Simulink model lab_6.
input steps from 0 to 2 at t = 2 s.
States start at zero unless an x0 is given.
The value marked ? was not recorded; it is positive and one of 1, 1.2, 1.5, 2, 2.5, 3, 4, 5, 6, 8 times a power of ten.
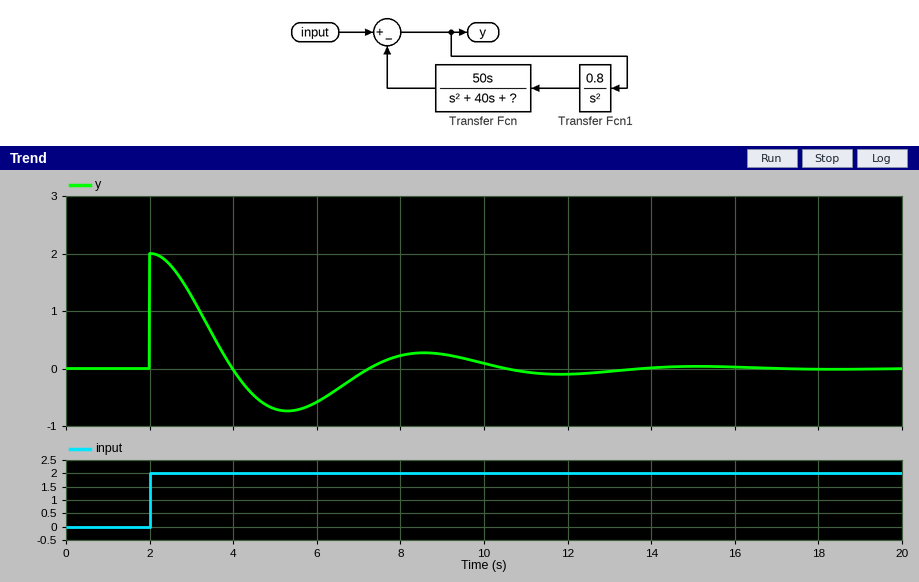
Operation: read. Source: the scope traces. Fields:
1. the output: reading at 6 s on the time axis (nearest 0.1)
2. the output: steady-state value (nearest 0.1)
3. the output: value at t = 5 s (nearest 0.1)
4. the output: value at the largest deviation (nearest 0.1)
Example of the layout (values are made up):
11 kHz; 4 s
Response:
-0.6; 0.0; -0.7; 2.0
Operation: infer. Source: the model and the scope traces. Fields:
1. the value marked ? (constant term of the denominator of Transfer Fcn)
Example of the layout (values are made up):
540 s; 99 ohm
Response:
25
